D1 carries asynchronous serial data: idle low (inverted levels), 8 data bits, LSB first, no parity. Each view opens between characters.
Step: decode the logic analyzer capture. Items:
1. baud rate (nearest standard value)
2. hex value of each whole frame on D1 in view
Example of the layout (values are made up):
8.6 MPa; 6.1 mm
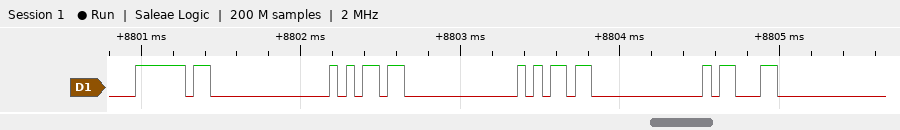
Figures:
19200 baud; 20, 25, 25, 39
